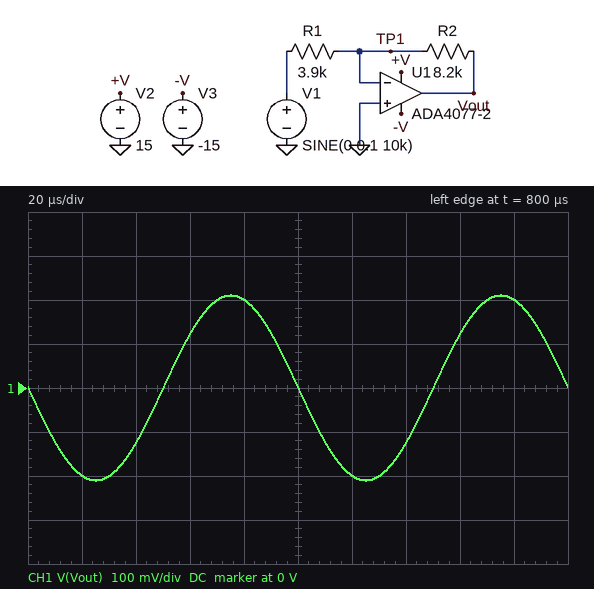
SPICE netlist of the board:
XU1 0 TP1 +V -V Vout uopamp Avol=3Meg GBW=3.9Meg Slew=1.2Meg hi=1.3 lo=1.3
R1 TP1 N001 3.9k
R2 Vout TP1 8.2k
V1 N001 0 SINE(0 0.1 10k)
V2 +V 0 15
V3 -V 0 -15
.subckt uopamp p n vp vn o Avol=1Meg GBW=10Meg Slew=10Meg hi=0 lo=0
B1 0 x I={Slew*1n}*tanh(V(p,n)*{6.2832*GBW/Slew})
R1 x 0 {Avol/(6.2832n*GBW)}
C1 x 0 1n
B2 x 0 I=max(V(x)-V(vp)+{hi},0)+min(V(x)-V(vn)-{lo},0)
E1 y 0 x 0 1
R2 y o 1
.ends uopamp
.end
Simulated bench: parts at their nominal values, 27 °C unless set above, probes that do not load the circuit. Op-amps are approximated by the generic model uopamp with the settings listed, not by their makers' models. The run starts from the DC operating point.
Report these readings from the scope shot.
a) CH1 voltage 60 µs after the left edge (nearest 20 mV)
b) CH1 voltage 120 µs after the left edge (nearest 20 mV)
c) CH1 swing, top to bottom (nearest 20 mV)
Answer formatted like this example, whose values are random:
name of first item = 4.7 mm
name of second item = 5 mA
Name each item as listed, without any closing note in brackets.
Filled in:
CH1 voltage 60 µs after the left edge = 120 mV
CH1 voltage 120 µs after the left edge = -200 mV
CH1 swing, top to bottom = 420 mV
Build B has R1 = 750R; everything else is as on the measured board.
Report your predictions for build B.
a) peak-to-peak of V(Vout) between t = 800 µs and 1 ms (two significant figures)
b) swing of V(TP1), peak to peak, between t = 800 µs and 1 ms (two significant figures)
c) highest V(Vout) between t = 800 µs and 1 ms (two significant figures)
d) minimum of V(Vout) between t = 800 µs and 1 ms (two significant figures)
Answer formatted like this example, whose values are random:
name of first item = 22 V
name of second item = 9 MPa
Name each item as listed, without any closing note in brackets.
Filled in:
peak-to-peak of V(Vout) between t = 800 µs and 1 ms = 2.2 V
swing of V(TP1), peak to peak, between t = 800 µs and 1 ms = 5.6 mV
highest V(Vout) between t = 800 µs and 1 ms = 1.1 V
minimum of V(Vout) between t = 800 µs and 1 ms = -1.1 V
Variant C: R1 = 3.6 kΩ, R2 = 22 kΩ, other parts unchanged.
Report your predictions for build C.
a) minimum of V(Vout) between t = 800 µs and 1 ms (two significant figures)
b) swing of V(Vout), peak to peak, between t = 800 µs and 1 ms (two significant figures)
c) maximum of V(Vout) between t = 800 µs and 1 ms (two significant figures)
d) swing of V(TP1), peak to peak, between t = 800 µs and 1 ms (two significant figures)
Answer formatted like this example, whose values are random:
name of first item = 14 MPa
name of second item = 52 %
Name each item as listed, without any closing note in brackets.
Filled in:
minimum of V(Vout) between t = 800 µs and 1 ms = -610 mV
swing of V(Vout), peak to peak, between t = 800 µs and 1 ms = 1.2 V
maximum of V(Vout) between t = 800 µs and 1 ms = 610 mV
swing of V(TP1), peak to peak, between t = 800 µs and 1 ms = 3.1 mV
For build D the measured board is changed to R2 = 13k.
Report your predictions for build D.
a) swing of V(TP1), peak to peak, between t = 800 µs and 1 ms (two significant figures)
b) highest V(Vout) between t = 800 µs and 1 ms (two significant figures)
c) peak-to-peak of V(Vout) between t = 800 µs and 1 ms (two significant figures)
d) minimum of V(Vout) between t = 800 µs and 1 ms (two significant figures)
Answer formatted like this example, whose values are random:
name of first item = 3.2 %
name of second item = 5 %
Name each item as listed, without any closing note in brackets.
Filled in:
swing of V(TP1), peak to peak, between t = 800 µs and 1 ms = 1.7 mV
highest V(Vout) between t = 800 µs and 1 ms = 330 mV
peak-to-peak of V(Vout) between t = 800 µs and 1 ms = 670 mV
minimum of V(Vout) between t = 800 µs and 1 ms = -330 mV
